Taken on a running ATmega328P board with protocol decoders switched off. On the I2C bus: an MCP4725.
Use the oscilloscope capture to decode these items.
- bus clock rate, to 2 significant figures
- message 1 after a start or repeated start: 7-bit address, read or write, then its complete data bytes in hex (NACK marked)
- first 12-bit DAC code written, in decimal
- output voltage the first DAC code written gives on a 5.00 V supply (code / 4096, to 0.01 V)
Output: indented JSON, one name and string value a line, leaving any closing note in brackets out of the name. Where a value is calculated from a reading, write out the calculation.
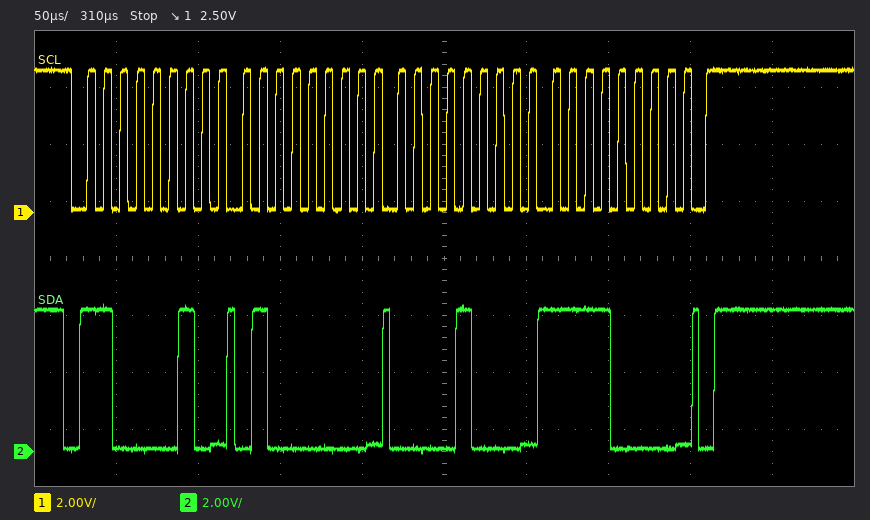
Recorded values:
{
  "bus clock rate, to 2 significant figures": "100 kHz",
  "message 1 after a start or repeated start: 7-bit address, read or write, then its complete data bytes in hex": "0x61 write: 40 08 F0",
  "first 12-bit DAC code written, in decimal": "143",
  "output voltage the first DAC code written gives on a 5.00 V supply": "143 / 4096 x 5.00 V = 0.17 V"
}
